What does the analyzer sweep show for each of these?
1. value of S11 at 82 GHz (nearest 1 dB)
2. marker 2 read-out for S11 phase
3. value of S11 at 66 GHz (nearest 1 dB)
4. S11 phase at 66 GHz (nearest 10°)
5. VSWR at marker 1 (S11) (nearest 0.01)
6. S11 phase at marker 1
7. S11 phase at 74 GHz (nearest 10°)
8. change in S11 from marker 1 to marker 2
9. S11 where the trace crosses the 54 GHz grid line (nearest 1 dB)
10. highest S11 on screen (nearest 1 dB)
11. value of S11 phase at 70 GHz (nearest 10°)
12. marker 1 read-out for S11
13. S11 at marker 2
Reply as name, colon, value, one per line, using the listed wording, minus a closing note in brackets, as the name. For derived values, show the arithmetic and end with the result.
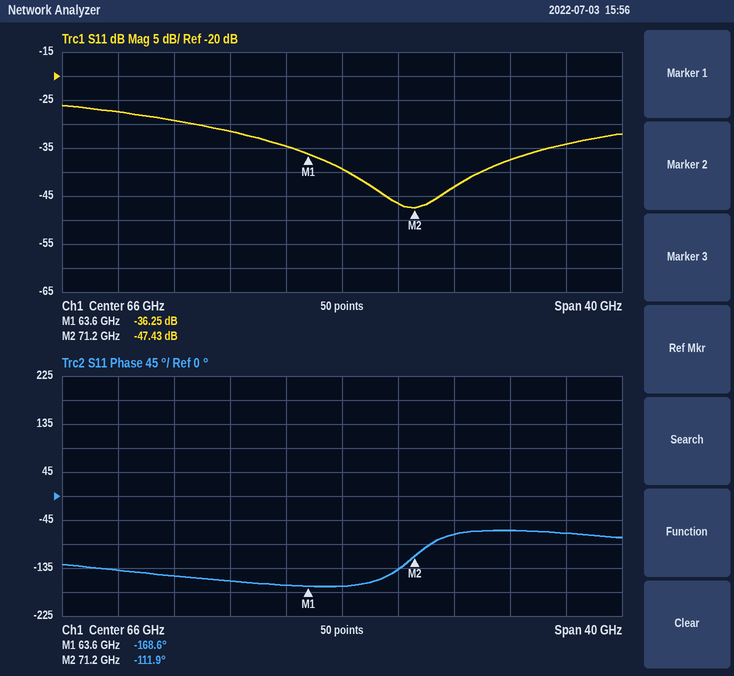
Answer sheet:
value of S11 at 82 GHz: -34 dB
marker 2 read-out for S11 phase: -111.9°
value of S11 at 66 GHz: -39 dB
S11 phase at 66 GHz: -170°
VSWR at marker 1 (S11): (1 + 0.0154)/(1 − 0.0154) ≈ 1.03
S11 phase at marker 1: -168.6°
S11 phase at 74 GHz: -70°
change in S11 from marker 1 to marker 2: -47.43 − (-36.25) = -11.18 dB
S11 where the trace crosses the 54 GHz grid line: -29 dB
highest S11 on screen: -26 dB
value of S11 phase at 70 GHz: -140°
marker 1 read-out for S11: -36.25 dB
S11 at marker 2: -47.43 dB
